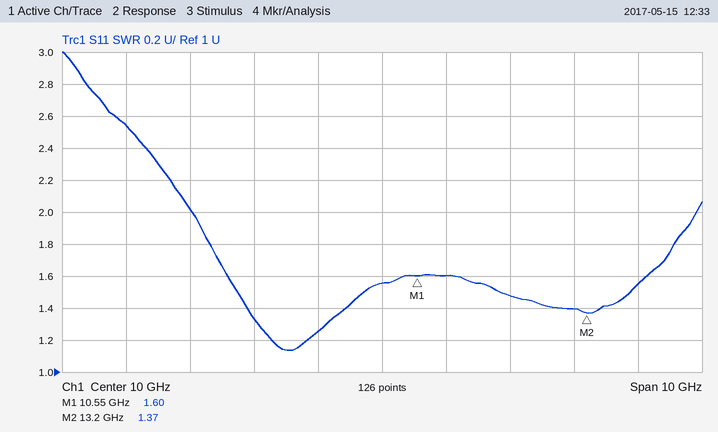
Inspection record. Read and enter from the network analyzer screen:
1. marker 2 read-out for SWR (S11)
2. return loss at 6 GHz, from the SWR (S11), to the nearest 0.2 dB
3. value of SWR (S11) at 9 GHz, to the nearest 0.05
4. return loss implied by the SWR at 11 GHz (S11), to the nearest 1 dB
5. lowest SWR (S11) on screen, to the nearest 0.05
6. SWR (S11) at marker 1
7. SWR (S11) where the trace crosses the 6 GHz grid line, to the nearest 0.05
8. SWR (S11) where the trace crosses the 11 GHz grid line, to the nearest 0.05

1.37
7.2 dB
1.25
13 dB
1.15
1.60
2.55
1.60
